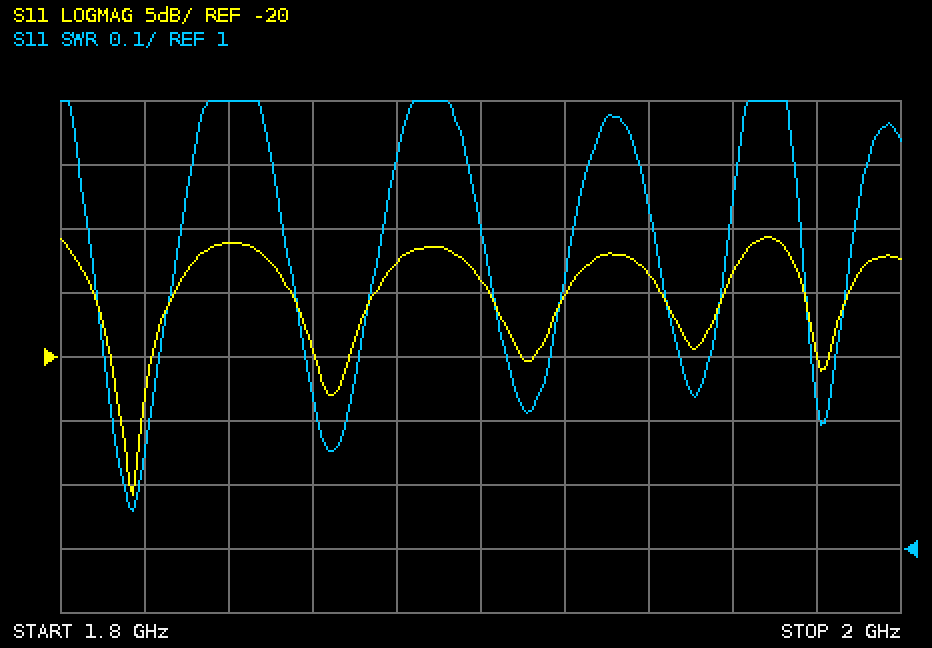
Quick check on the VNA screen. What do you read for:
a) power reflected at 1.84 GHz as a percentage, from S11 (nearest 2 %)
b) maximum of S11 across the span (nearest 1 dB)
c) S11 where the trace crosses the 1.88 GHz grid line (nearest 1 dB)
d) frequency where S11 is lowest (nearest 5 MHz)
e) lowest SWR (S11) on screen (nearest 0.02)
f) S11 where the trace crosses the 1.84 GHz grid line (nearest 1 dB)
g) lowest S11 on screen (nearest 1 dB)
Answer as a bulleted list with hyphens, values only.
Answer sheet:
- 8 %
- -11 dB
- -13 dB
- 1.815 GHz
- 1.06
- -11 dB
- -31 dB
